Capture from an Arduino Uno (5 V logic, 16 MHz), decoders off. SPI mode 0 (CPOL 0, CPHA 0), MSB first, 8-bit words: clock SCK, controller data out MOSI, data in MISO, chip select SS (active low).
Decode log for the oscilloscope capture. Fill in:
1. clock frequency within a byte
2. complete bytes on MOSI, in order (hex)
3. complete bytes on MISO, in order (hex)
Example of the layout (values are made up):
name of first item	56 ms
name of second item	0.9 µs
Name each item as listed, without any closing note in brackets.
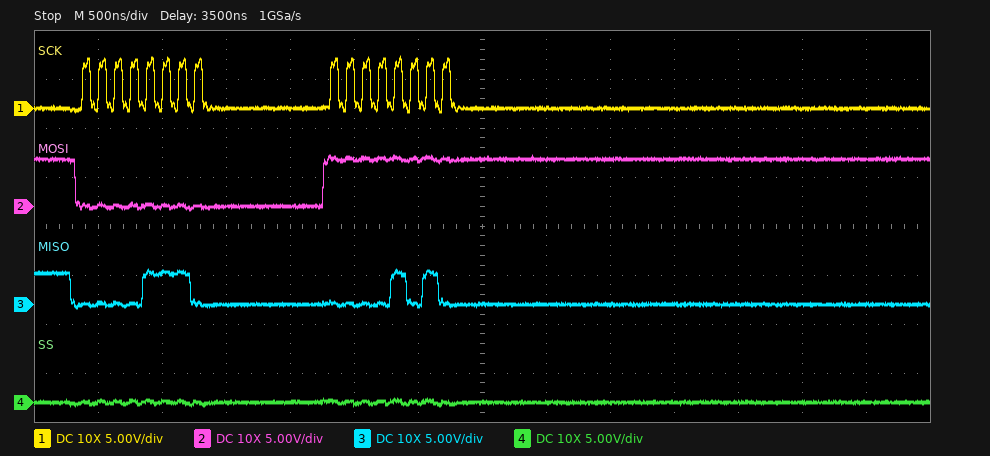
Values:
clock frequency within a byte	8 MHz
complete bytes on MOSI, in order	00 FF
complete bytes on MISO, in order	0E 0A
